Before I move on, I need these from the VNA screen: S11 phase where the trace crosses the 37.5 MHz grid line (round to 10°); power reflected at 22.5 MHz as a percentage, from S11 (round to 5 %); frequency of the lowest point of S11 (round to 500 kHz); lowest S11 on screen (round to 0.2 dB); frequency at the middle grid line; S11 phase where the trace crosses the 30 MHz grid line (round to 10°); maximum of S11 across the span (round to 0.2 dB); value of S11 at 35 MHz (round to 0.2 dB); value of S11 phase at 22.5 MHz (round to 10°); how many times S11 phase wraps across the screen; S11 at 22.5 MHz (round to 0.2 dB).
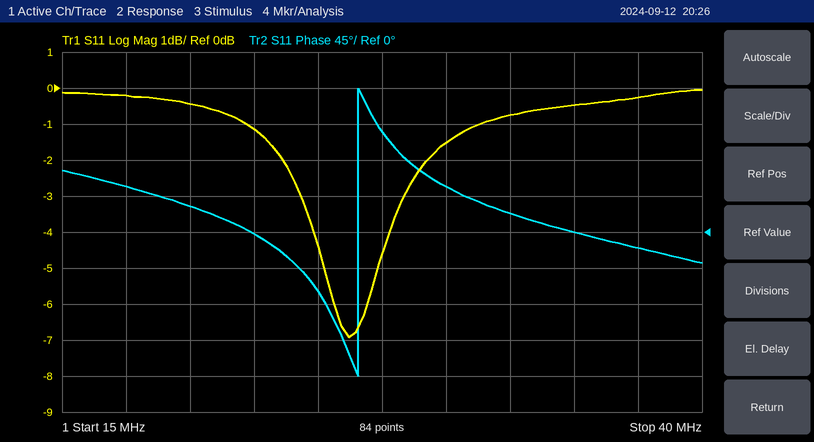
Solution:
-20°
75 %
26.0 MHz
-7.0 dB
27.5 MHz
60°
0.0 dB
-0.4 dB
0°
1
-1.2 dB
